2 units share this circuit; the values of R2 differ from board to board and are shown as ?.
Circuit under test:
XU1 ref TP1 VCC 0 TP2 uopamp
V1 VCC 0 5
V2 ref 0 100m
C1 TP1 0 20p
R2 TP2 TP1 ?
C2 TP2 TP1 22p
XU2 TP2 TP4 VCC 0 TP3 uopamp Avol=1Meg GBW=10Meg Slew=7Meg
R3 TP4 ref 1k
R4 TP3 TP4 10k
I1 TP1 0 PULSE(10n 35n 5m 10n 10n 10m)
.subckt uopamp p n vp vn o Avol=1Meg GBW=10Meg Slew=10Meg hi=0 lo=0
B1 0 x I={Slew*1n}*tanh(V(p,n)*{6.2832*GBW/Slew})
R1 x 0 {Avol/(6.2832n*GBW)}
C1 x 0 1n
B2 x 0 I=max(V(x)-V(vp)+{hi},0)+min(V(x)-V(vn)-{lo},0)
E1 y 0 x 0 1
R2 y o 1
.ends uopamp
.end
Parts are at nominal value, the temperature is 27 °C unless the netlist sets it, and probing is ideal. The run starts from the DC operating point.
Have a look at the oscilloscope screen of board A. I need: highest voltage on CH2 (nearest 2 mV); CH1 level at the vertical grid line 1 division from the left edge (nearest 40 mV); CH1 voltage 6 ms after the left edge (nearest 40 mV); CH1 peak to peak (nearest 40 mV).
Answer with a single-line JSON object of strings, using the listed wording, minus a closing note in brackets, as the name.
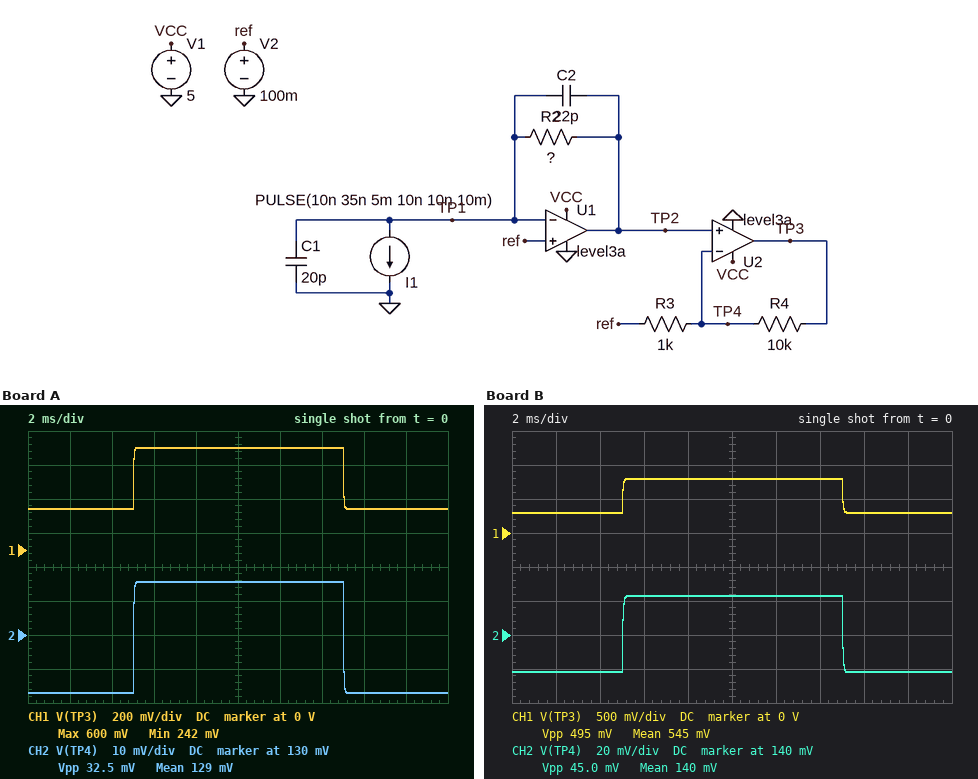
{"highest voltage on CH2": "146 mV", "CH1 level at the vertical grid line 1 division from the left edge": "240 mV", "CH1 voltage 6 ms after the left edge": "600 mV", "CH1 peak to peak": "360 mV"}
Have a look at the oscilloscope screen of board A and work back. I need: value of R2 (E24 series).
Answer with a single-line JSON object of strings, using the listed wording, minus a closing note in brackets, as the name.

{"value of R2": "1.3 MΩ"}
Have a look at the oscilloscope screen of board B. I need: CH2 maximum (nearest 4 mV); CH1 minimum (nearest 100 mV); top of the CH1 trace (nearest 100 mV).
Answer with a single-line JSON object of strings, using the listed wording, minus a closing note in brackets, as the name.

{"CH2 maximum": "164 mV", "CH1 minimum": "300 mV", "top of the CH1 trace": "800 mV"}
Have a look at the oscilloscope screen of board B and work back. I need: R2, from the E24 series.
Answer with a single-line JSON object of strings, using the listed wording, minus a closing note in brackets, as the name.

{"R2, from the E24 series": "1.8 MΩ"}
